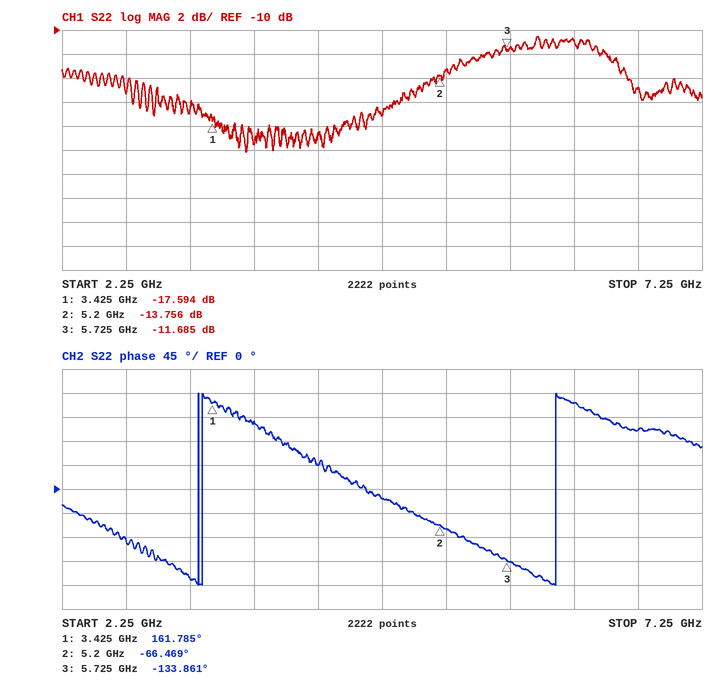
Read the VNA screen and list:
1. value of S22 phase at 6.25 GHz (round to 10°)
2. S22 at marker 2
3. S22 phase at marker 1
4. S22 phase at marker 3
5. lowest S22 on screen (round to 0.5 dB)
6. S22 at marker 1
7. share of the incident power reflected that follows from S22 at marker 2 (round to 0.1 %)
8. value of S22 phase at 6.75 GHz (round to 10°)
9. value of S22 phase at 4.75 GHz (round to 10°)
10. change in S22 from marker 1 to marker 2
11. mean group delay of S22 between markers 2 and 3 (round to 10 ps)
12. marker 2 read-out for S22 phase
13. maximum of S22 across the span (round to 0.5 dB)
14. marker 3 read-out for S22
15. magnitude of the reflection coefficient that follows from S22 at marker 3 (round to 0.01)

160°
-13.756 dB
161.785°
-133.861°
-20.0 dB
-17.594 dB
4.2 %
110°
-20°
3.838 dB
360 ps
-66.469°
-10.5 dB
-11.685 dB
0.26
